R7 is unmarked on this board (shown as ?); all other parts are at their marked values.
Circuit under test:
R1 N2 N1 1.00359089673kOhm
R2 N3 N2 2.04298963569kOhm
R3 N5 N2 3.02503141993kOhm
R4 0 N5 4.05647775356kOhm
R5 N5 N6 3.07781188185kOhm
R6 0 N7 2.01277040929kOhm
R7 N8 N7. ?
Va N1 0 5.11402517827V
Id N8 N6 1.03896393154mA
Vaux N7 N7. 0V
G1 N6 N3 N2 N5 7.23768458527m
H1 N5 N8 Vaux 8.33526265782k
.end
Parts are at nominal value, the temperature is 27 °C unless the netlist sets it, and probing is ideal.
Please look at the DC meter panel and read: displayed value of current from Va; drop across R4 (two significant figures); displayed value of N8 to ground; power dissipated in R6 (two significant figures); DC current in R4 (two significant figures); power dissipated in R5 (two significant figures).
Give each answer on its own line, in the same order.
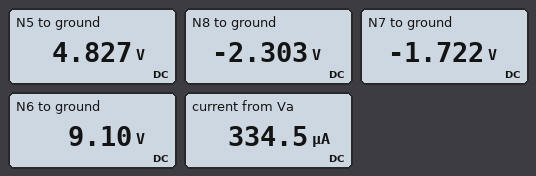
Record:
334.5 µA
4.8 V
-2.303 V
1.5 mW
1.2 mA
5.9 mW
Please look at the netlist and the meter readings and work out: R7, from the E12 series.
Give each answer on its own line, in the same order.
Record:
680 Ω
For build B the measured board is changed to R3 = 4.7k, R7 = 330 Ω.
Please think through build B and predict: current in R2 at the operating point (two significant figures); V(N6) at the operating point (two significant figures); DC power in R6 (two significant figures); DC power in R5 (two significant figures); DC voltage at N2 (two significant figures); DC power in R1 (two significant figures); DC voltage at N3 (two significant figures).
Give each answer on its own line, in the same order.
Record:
390 µA
9.2 V
1.3 mW
6.3 mW
4.7 V
150 µW
3.9 V
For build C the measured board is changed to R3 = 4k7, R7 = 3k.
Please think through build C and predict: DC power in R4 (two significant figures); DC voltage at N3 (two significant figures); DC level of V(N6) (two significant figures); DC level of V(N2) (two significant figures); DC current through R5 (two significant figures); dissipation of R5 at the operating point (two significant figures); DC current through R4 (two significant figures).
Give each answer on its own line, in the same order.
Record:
7.1 mW
6.0 V
7.6 V
5.4 V
740 µA
1.7 mW
1.3 mA
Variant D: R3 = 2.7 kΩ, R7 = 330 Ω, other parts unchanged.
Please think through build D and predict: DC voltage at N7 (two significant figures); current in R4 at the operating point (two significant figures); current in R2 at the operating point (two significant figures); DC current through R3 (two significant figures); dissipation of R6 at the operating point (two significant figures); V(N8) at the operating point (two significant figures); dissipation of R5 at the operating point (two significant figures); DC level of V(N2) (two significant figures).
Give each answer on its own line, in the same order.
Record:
-1.6 V
1.2 mA
400 µA
21 µA
1.3 mW
-1.9 V
6.4 mW
4.7 V
